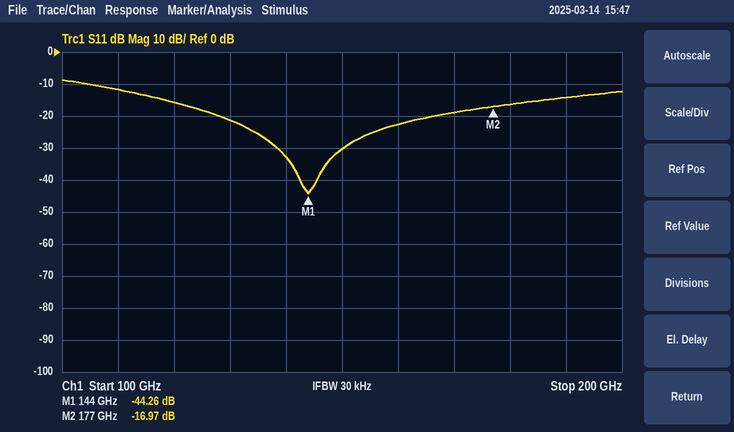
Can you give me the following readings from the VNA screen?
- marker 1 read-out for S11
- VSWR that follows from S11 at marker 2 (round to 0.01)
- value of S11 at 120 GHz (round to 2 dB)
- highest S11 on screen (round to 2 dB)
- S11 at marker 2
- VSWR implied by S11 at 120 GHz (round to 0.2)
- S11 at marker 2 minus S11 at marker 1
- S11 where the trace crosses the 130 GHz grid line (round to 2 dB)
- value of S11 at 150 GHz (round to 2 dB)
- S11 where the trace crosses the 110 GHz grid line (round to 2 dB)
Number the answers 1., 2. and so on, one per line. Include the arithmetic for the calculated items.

1. -44.26 dB
2. (1 + 0.1417)/(1 − 0.1417) ≈ 1.33
3. -16 dB
4. -8 dB
5. -16.97 dB
6. |Γ| = 10^(-16/20) = 0.1585; VSWR = (1 + 0.1585)/(1 − 0.1585) ≈ 1.4
7. -16.97 − (-44.26) = 27.29 dB
8. -22 dB
9. -30 dB
10. -12 dB
